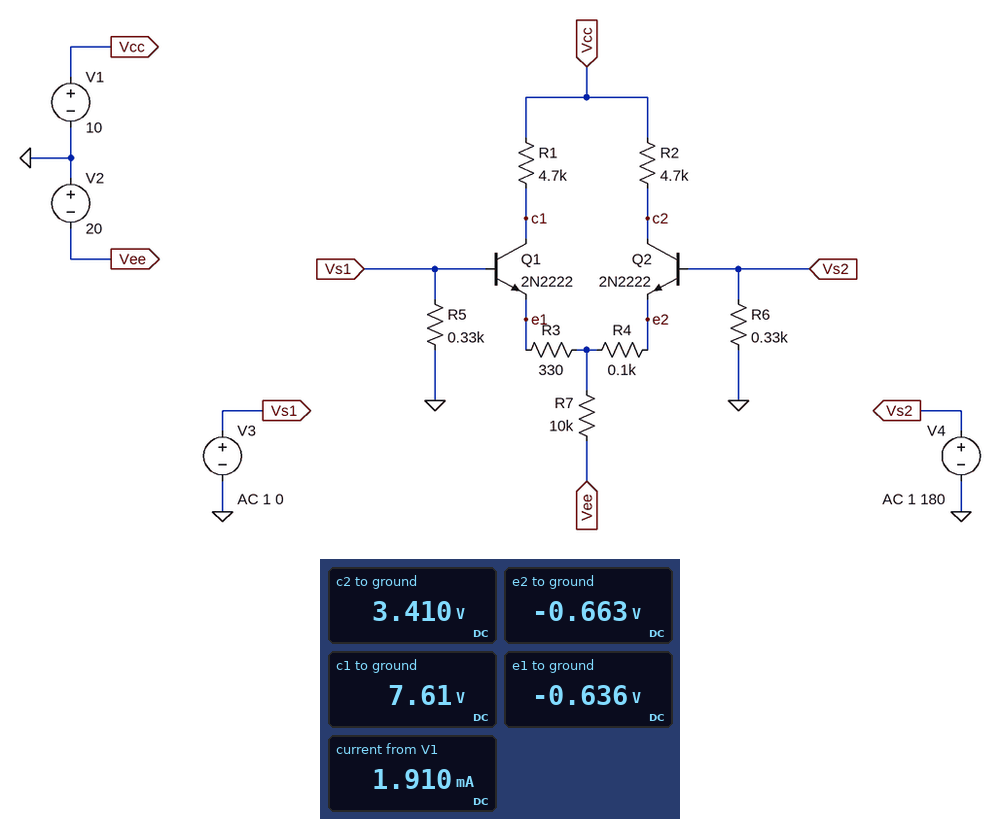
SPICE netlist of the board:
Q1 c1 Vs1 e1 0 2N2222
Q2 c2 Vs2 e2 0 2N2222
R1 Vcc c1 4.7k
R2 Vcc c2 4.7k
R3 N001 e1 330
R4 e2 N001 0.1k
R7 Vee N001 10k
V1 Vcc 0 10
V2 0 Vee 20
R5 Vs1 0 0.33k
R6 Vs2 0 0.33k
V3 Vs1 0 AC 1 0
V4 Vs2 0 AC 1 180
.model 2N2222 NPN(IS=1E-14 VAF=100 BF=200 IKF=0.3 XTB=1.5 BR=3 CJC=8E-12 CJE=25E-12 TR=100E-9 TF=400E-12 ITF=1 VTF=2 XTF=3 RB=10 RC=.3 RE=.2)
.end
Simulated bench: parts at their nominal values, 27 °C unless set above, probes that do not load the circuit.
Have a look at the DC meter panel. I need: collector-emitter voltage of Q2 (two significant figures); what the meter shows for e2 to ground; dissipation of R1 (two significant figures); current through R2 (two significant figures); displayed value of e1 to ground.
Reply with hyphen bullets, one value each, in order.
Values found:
- 4.1 V
- -0.663 V
- 1.2 mW
- 1.4 mA
- -0.636 V
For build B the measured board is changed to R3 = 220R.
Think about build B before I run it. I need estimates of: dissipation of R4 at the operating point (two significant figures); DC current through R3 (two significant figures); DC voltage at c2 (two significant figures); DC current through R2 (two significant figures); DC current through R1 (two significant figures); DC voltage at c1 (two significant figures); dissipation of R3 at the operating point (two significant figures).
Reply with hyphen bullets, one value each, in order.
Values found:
- 160 µW
- 660 µA
- 4.1 V
- 1.3 mA
- 650 µA
- 6.9 V
- 95 µW
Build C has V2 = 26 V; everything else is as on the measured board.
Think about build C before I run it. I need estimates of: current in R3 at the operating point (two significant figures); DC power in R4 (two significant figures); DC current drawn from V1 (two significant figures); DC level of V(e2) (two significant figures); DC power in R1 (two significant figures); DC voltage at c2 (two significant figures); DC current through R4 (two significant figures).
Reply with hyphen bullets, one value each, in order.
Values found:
- 650 µA
- 350 µW
- 2.5 mA
- -670 mV
- 2.0 mW
- 1.3 V
- 1.9 mA
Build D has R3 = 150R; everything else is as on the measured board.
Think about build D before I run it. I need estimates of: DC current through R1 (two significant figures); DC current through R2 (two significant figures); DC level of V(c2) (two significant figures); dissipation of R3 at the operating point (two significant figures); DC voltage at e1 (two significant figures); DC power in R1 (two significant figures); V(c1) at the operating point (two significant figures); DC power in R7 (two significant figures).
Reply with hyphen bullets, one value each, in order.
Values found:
- 800 µA
- 1.1 mA
- 4.8 V
- 97 µW
- -650 mV
- 3.0 mW
- 6.2 V
- 37 mW
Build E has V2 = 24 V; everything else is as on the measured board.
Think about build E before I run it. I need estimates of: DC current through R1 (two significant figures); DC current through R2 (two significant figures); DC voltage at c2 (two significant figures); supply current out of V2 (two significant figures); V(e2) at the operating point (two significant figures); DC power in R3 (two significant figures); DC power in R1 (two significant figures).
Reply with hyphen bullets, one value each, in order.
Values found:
- 600 µA
- 1.7 mA
- 2.0 V
- 2.3 mA
- -670 mV
- 120 µW
- 1.7 mW
